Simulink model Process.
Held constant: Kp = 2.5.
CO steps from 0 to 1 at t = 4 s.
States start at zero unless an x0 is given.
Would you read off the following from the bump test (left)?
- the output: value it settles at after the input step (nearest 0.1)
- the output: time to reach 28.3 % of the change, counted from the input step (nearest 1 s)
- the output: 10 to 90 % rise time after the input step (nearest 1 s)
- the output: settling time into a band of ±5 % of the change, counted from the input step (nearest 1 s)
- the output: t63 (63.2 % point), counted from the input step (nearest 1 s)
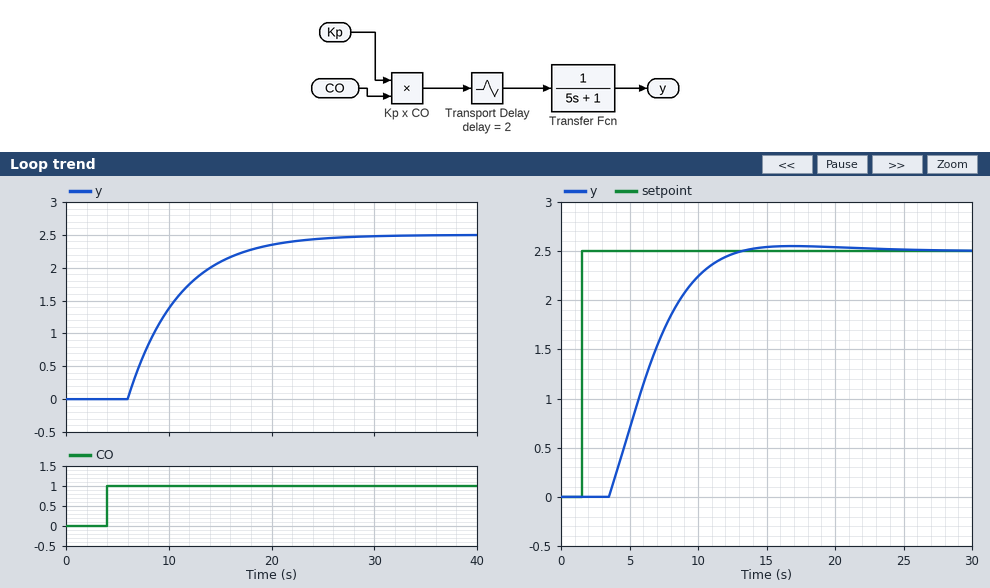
2.5
4 s
11 s
17 s
7 s
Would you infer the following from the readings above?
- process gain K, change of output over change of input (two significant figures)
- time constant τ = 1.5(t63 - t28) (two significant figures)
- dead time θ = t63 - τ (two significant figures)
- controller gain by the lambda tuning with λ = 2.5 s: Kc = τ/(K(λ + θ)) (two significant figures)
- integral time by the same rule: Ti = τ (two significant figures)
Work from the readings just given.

2.5
4.5 s
2.5 s
0.36
4.5 s
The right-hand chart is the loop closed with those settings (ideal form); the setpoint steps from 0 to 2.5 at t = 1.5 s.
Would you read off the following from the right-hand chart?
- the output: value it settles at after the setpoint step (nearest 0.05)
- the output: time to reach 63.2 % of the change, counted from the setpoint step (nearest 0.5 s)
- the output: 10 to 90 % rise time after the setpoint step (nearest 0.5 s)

2.50
5.5 s
6.0 s
